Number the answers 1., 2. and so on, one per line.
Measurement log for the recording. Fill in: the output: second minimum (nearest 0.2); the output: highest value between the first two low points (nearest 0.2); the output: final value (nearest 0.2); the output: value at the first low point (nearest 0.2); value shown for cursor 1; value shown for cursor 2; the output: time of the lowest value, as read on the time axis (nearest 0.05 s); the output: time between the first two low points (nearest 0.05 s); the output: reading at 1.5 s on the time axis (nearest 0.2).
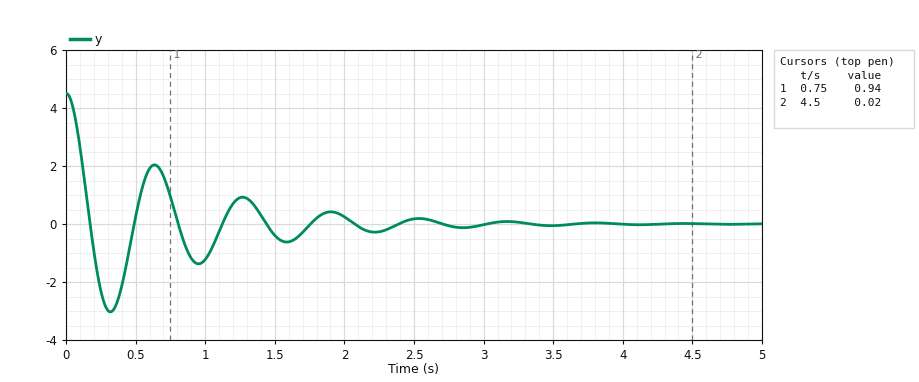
1. -1.4
2. 2.0
3. 0.0
4. -3.0
5. 0.94
6. 0.02
7. 0.30 s
8. 0.65 s
9. -0.4
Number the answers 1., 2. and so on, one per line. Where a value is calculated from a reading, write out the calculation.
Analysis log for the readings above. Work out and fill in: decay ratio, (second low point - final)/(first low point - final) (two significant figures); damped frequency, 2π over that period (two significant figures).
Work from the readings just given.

1. (-1.4 - 0) / (-3 - 0) = 0.47
2. 2π / 0.65 = 9.7 rad/s
